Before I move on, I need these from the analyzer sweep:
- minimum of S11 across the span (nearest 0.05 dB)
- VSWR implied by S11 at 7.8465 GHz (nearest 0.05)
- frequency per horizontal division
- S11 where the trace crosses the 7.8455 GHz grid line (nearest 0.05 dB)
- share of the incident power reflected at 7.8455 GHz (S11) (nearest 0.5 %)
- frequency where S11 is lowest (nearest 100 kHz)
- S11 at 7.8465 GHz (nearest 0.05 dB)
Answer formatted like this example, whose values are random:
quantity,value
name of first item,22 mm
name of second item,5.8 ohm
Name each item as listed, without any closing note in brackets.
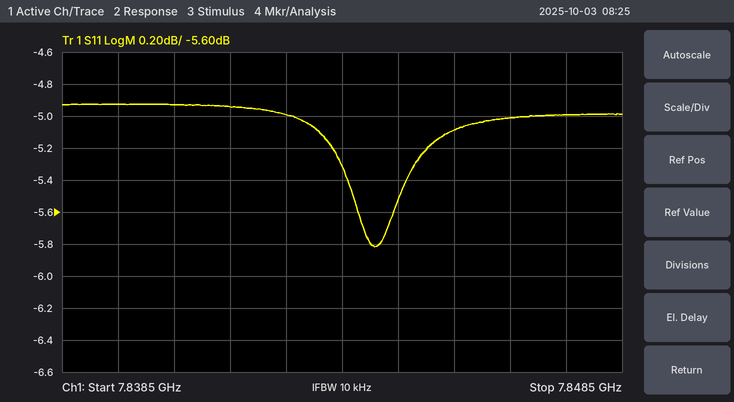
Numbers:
quantity,value
minimum of S11 across the span,-5.80 dB
VSWR implied by S11 at 7.8465 GHz,3.55
frequency per horizontal division,1 MHz
S11 where the trace crosses the 7.8455 GHz grid line,-5.10 dB
share of the incident power reflected at 7.8455 GHz (S11),31.0 %
frequency where S11 is lowest,7.8441 GHz
S11 at 7.8465 GHz,-5.00 dB
